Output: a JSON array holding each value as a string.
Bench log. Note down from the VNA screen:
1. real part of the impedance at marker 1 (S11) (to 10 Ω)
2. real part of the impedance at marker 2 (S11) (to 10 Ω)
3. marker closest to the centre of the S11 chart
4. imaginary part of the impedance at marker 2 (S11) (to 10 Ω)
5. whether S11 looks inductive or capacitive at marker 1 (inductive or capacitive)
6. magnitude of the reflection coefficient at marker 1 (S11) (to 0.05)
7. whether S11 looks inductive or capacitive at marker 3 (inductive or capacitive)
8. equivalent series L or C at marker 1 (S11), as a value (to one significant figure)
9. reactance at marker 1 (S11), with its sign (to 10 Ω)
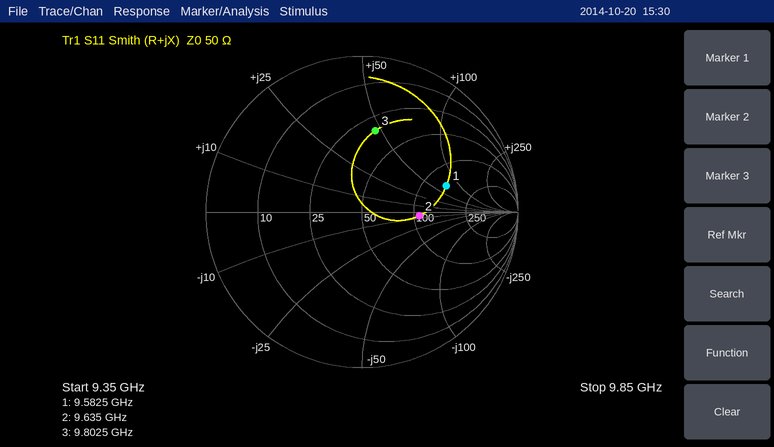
["140 Ω", "110 Ω", "marker 2", "-10 Ω", "inductive", "0.55", "inductive", "1 nH", "+70 Ω"]
